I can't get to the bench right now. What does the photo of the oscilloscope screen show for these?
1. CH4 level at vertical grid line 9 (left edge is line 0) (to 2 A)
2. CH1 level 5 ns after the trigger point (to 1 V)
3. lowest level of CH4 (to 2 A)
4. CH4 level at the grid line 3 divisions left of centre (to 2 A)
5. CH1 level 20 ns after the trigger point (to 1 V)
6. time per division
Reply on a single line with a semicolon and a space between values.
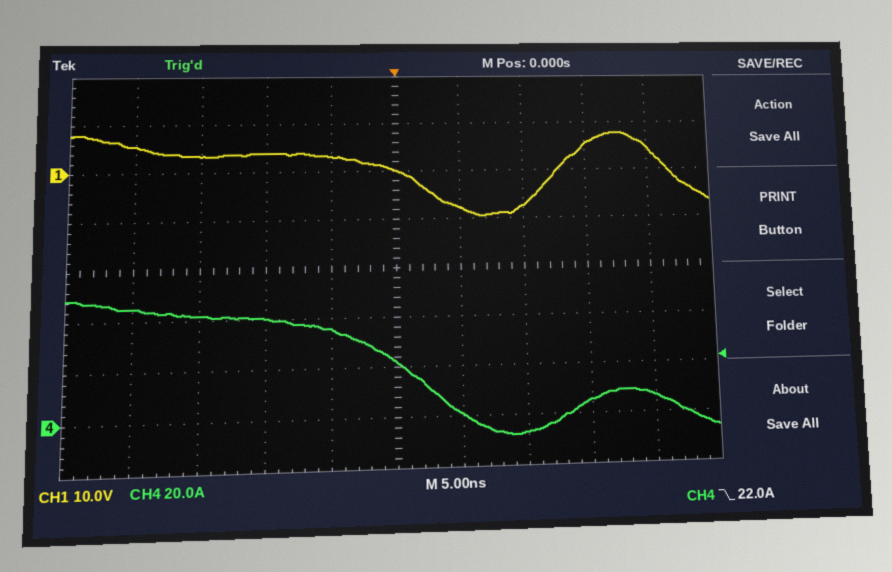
6 A; -8 V; -8 A; 42 A; 5 V; 5 ns
